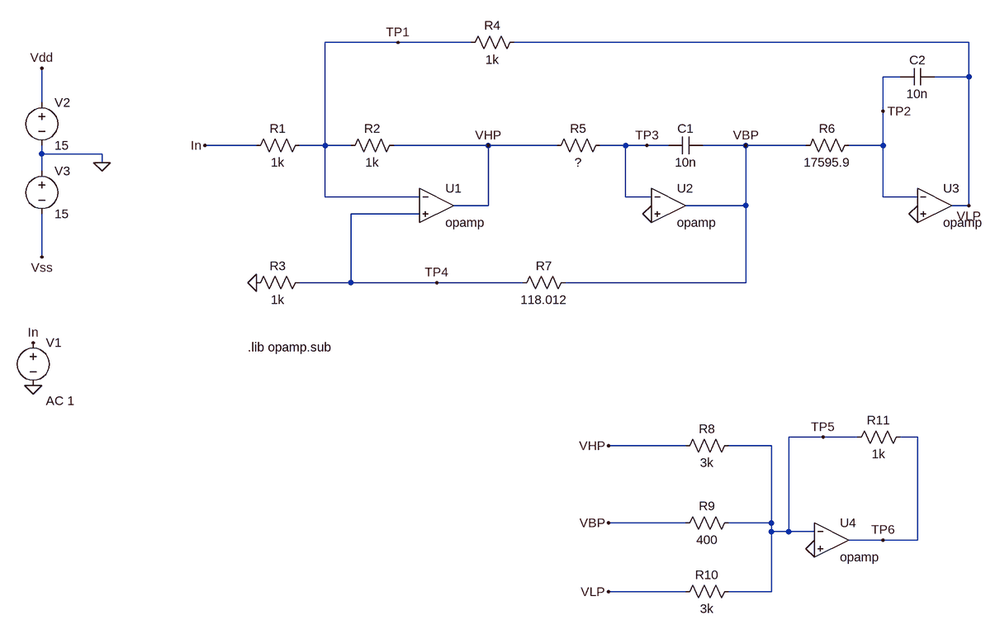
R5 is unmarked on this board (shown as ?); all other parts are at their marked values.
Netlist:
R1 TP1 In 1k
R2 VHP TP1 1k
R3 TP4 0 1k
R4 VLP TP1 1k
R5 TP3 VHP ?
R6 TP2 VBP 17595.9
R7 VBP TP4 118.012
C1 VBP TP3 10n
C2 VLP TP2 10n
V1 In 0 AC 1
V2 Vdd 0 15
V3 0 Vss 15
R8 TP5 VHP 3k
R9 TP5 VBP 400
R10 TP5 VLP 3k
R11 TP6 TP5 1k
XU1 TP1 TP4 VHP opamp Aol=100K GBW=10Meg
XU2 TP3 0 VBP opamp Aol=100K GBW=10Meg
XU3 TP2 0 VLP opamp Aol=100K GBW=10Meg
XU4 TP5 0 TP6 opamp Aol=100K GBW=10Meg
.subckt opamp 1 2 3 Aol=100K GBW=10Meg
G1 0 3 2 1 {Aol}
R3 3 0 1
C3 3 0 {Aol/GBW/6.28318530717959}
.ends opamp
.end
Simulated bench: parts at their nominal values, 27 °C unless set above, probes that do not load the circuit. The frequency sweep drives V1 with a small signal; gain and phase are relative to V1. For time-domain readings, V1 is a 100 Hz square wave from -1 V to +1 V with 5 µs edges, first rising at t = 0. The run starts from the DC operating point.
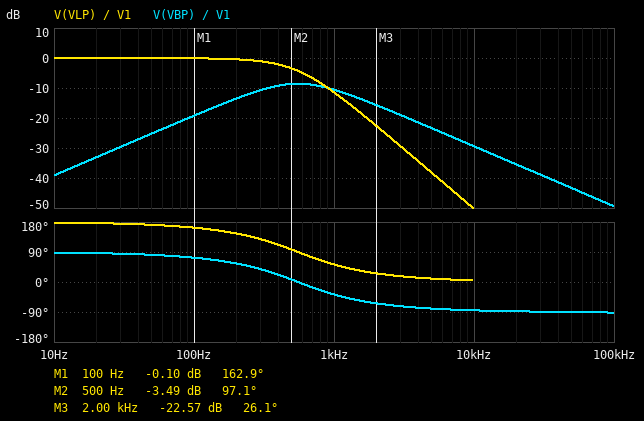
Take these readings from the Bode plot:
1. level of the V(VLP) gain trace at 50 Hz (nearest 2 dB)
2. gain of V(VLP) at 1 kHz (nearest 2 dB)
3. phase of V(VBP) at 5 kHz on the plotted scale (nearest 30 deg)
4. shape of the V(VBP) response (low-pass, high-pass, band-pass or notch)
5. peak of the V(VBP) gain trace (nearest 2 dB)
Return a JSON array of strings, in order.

["0 dB", "-12 dB", "-90 deg", "band-pass", "-8 dB"]
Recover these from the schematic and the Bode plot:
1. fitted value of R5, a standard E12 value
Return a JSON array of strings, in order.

["47 kΩ"]
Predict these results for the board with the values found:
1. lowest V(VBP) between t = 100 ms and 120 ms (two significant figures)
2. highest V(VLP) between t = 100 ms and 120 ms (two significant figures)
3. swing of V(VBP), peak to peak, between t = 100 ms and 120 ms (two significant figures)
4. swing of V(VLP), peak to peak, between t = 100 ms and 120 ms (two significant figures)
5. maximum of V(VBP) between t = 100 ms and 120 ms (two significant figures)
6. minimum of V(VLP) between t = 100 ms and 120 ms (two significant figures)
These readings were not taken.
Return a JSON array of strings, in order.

["-510 mV", "1.0 V", "1.0 V", "2.0 V", "510 mV", "-1.0 V"]
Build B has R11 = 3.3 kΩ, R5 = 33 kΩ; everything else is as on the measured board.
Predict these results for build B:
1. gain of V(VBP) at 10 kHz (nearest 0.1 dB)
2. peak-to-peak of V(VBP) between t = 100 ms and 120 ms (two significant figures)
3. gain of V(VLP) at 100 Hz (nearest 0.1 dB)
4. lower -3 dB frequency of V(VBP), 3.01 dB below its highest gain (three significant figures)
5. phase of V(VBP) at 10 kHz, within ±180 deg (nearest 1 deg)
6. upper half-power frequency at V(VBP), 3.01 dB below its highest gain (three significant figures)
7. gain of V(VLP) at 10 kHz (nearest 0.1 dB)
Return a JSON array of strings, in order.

["-26.4 dB", "1.1 V", "-0.2 dB", "278 Hz", "-83 deg", "1.57 kHz", "-47.2 dB"]
